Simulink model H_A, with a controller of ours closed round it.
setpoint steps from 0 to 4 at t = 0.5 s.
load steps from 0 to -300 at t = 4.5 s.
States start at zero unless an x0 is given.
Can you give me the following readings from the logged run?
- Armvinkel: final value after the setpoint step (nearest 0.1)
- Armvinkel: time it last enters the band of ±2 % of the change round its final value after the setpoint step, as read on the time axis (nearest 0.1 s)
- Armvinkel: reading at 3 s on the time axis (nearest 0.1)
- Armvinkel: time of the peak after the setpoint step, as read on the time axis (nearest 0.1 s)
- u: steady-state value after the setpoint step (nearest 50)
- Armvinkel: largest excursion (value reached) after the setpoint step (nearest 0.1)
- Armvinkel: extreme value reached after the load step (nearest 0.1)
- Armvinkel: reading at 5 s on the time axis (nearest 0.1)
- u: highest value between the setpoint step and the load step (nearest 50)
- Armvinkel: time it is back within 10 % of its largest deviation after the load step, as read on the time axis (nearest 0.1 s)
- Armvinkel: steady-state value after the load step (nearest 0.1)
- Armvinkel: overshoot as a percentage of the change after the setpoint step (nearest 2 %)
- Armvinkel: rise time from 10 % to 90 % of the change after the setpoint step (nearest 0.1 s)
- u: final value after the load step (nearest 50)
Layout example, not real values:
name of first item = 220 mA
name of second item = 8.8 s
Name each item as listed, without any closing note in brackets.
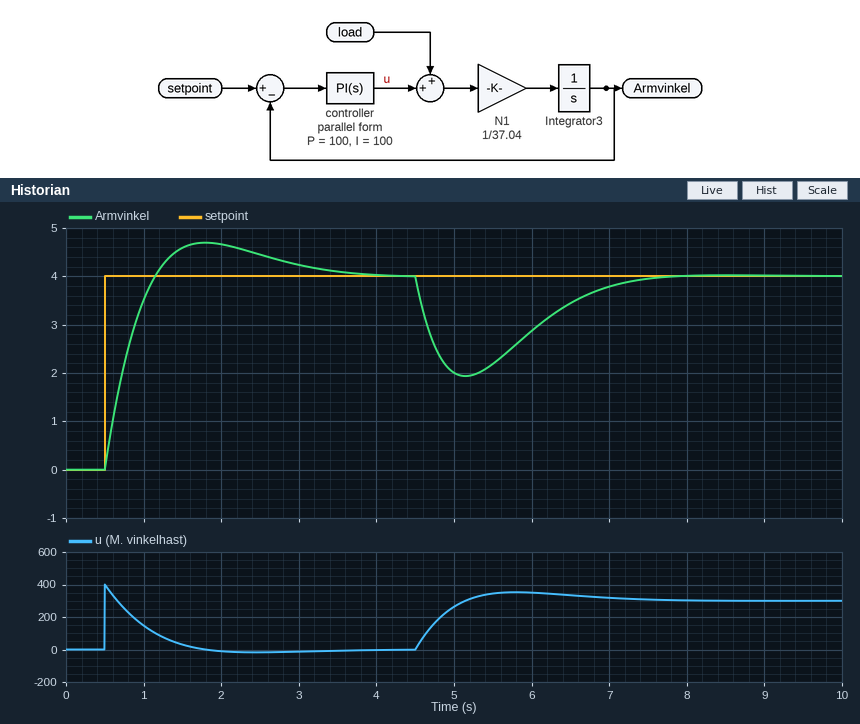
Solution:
Armvinkel: final value after the setpoint step = 4.0
Armvinkel: time it last enters the band of ±2 % of the change round its final value after the setpoint step, as read on the time axis = 3.6 s
Armvinkel: reading at 3 s on the time axis = 4.2
Armvinkel: time of the peak after the setpoint step, as read on the time axis = 1.8 s
u: steady-state value after the setpoint step = 0
Armvinkel: largest excursion (value reached) after the setpoint step = 4.7
Armvinkel: extreme value reached after the load step = 1.9
Armvinkel: reading at 5 s on the time axis = 2.0
u: highest value between the setpoint step and the load step = 400
Armvinkel: time it is back within 10 % of its largest deviation after the load step, as read on the time axis = 7.0 s
Armvinkel: steady-state value after the load step = 4.0
Armvinkel: overshoot as a percentage of the change after the setpoint step = 18 %
Armvinkel: rise time from 10 % to 90 % of the change after the setpoint step = 0.5 s
u: final value after the load step = 300
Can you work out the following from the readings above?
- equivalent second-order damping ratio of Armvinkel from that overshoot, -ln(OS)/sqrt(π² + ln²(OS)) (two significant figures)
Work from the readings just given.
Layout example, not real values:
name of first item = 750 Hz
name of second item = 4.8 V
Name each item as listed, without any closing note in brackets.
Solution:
equivalent second-order damping ratio of Armvinkel from that overshoot, -ln(OS)/sqrt(π² + ln²(OS)) = 0.48
